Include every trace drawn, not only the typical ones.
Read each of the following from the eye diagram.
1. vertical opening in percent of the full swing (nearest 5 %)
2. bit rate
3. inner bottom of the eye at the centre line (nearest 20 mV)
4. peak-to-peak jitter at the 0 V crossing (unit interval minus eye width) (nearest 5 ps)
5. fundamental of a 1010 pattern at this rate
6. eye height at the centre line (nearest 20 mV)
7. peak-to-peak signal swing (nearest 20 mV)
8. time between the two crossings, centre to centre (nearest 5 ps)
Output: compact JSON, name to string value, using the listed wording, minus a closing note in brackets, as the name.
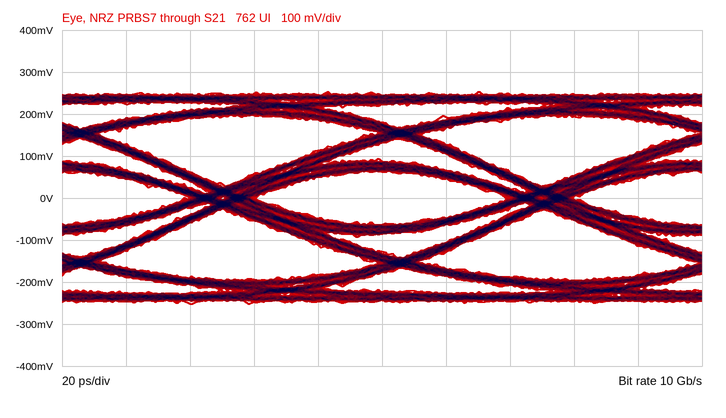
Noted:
{"vertical opening in percent of the full swing": "25 %", "bit rate": "10 Gb/s", "inner bottom of the eye at the centre line": "-60 mV", "peak-to-peak jitter at the 0 V crossing (unit interval minus eye width)": "20 ps", "fundamental of a 1010 pattern at this rate": "5 GHz", "eye height at the centre line": "120 mV", "peak-to-peak signal swing": "500 mV", "time between the two crossings, centre to centre": "100 ps"}
